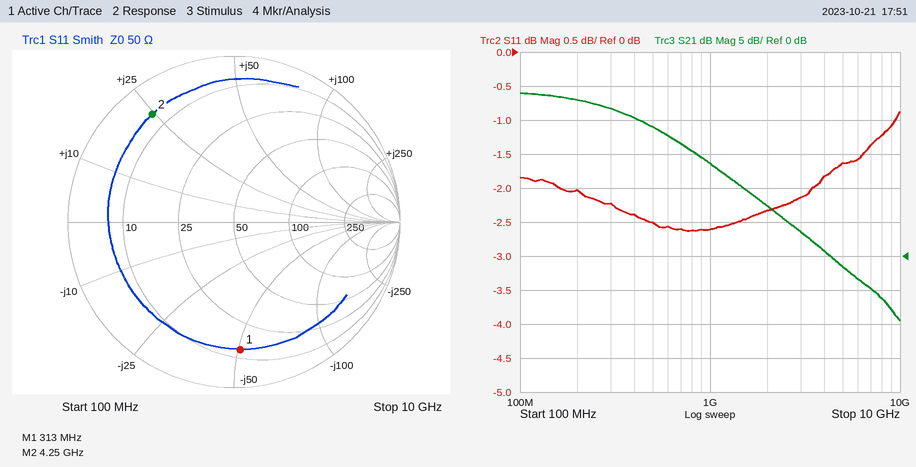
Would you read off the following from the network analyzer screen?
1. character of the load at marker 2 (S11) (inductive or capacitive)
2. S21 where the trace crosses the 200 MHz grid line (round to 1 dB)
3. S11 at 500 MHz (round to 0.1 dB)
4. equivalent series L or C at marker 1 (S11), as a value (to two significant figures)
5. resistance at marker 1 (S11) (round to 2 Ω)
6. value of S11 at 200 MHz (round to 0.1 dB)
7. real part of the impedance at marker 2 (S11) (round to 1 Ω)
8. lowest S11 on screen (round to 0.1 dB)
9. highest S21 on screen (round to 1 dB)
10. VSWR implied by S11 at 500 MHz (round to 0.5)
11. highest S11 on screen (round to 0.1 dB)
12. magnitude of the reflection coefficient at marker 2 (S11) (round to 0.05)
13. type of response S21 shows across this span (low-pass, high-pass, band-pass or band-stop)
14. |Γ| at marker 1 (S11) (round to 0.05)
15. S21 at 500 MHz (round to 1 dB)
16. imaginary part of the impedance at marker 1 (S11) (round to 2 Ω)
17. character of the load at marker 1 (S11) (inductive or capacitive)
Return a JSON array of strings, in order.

["inductive", "23 dB", "-2.5 dB", "10 pF", "14 Ω", "-2.0 dB", "6 Ω", "-2.6 dB", "24 dB", "7.0", "-0.9 dB", "0.80", "low-pass", "0.75", "19 dB", "-50 Ω", "capacitive"]
